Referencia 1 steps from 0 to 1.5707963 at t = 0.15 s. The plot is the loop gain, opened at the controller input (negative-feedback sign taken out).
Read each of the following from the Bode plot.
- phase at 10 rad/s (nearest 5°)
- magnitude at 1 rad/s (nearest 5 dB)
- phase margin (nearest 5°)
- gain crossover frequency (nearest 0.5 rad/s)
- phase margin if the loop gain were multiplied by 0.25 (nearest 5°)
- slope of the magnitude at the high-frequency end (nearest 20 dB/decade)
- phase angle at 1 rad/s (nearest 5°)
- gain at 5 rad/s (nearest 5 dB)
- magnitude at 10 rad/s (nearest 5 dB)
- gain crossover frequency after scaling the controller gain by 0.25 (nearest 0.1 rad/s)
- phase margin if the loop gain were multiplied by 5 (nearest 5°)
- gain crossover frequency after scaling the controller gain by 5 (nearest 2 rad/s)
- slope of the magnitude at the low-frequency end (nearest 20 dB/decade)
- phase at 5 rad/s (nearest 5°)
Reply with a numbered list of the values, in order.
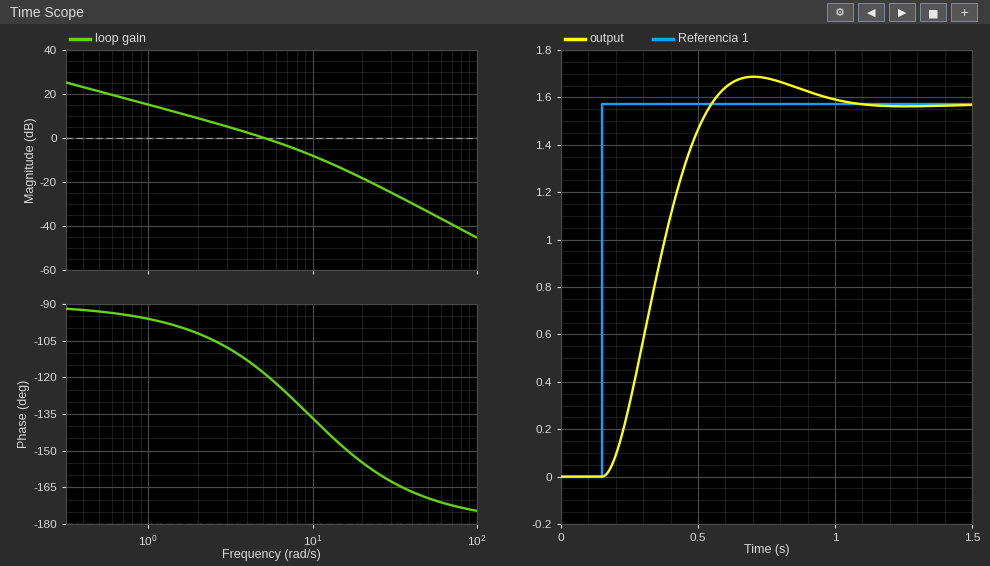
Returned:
1. -135°
2. 15 dB
3. 60°
4. 5.0 rad/s
5. 80°
6. -40 dB/decade
7. -95°
8. 0 dB
9. -10 dB
10. 1.4 rad/s
11. 30°
12. 16 rad/s
13. -20 dB/decade
14. -120°
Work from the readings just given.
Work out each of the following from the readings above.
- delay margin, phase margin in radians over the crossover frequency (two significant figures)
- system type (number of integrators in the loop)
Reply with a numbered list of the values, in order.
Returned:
1. 0.21 s
2. 1
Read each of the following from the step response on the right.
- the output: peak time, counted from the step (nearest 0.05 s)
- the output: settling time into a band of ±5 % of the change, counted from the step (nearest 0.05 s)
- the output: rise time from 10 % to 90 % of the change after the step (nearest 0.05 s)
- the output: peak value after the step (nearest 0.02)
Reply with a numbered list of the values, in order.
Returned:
1. 0.55 s
2. 0.70 s
3. 0.25 s
4. 1.68
